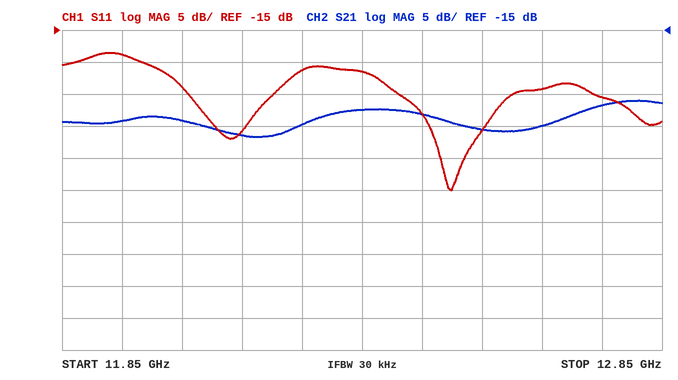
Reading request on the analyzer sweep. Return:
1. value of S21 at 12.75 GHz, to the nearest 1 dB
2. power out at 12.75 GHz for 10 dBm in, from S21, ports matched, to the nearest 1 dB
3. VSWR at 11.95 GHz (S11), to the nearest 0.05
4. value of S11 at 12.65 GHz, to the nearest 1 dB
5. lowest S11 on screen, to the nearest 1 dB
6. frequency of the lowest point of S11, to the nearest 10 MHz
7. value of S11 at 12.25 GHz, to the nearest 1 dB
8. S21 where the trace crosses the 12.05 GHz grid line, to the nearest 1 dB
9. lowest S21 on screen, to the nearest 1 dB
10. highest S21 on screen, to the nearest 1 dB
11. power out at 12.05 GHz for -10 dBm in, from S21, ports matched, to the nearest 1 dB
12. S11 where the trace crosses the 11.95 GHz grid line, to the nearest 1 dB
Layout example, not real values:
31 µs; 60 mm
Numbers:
-27 dB; -17 dBm; 1.25; -24 dB; -40 dB; 12.50 GHz; -21 dB; -29 dB; -32 dB; -26 dB; -39 dBm; -19 dB
